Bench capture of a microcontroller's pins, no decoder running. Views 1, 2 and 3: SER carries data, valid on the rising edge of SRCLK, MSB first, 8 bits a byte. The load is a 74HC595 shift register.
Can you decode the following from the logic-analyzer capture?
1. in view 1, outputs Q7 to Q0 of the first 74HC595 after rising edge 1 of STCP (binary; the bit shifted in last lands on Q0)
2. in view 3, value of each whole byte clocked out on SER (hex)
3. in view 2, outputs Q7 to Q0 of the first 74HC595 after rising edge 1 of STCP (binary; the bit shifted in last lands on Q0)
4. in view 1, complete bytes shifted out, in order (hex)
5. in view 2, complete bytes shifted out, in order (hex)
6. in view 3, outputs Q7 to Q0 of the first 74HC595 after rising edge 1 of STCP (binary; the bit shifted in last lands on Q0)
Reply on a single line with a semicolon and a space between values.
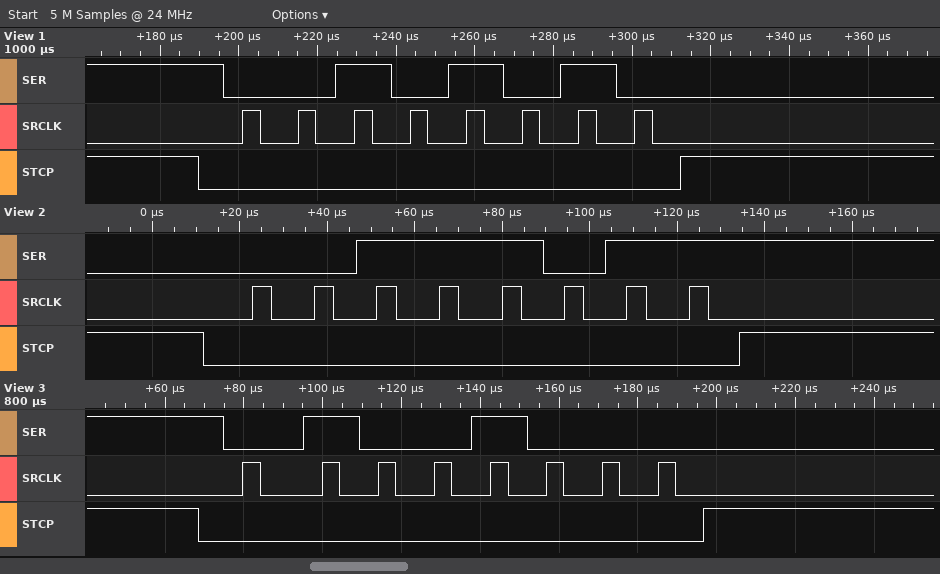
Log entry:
00101010; 48; 00111011; 2A; 0x3B; 01001000
